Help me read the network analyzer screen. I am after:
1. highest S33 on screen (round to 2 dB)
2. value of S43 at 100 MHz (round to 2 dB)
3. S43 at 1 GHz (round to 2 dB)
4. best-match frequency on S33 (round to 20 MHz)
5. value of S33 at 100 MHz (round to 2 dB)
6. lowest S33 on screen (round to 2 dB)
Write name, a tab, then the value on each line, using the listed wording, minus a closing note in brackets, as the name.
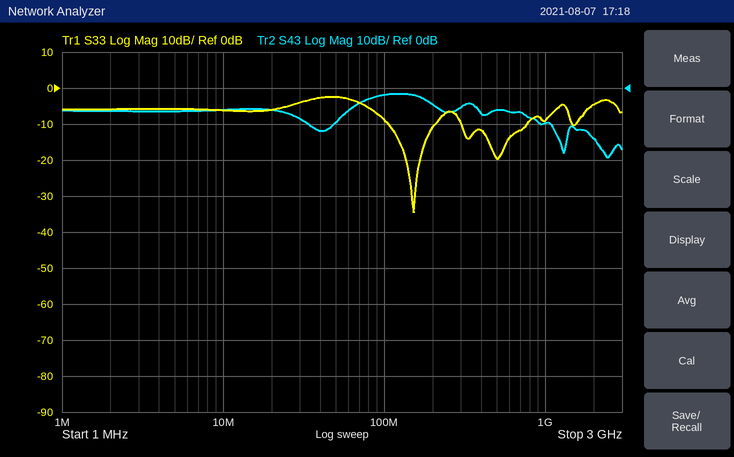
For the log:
highest S33 on screen	-2 dB
value of S43 at 100 MHz	-2 dB
S43 at 1 GHz	-10 dB
best-match frequency on S33	160 MHz
value of S33 at 100 MHz	-8 dB
lowest S33 on screen	-34 dB
